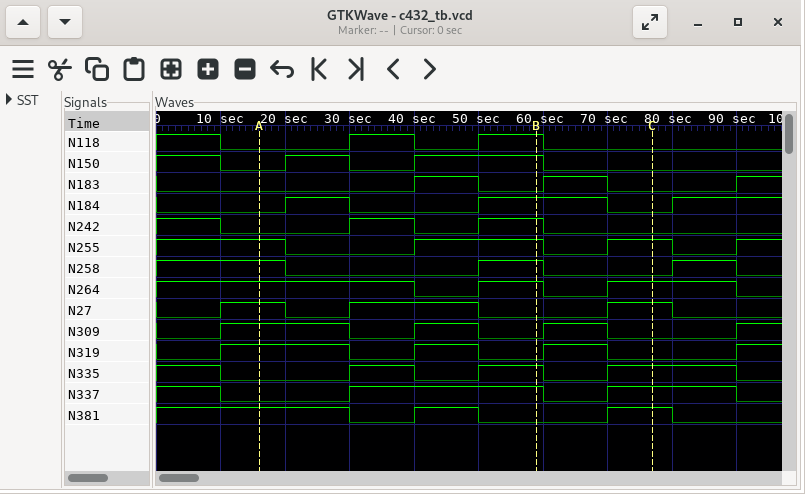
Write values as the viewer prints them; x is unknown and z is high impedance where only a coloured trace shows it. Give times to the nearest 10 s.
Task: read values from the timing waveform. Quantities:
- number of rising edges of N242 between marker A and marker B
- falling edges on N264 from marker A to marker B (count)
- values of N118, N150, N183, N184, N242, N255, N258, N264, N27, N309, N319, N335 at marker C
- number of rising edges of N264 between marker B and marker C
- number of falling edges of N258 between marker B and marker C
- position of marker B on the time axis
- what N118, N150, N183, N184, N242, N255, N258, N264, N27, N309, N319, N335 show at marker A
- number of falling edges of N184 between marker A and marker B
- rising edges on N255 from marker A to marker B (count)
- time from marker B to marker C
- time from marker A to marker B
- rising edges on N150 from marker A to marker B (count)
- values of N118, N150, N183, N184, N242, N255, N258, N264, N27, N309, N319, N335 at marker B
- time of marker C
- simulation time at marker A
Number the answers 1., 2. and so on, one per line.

1. 2
2. 1
3. N118=0, N150=0, N183=0, N184=0, N242=0, N255=1, N258=0, N264=1, N27=1, N309=0, N319=0, N335=1
4. 1
5. 1
6. 60 s
7. N118=0, N150=0, N183=0, N184=0, N242=0, N255=1, N258=1, N264=1, N27=1, N309=1, N319=1, N335=0
8. 1
9. 1
10. 20 s
11. 40 s
12. 2
13. N118=1, N150=1, N183=0, N184=1, N242=1, N255=1, N258=1, N264=1, N27=0, N309=0, N319=0, N335=1
14. 80 s
15. 20 s
